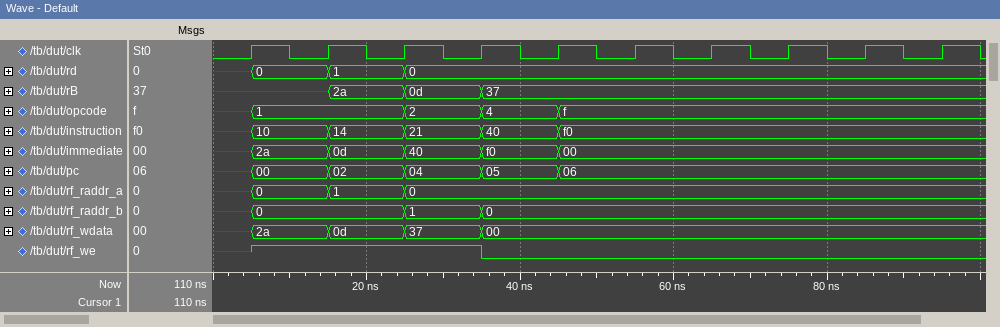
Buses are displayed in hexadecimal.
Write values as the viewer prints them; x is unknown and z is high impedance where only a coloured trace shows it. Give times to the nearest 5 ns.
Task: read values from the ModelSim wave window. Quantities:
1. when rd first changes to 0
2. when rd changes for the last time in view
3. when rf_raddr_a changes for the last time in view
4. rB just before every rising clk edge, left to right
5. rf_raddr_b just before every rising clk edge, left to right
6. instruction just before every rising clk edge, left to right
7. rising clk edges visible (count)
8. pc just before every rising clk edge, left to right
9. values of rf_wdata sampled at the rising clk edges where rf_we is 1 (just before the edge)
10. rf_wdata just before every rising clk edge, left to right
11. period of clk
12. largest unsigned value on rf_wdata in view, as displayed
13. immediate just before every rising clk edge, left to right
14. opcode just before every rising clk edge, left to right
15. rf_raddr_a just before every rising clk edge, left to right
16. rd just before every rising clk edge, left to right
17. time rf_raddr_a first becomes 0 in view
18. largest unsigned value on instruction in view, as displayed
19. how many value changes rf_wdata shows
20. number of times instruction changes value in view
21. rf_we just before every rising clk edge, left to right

5 ns
25 ns
25 ns
x, x, 2a, 0d, 37, 37, 37, 37, 37, 37
x, 0, 0, 1, 0, 0, 0, 0, 0, 0
x, 10, 14, 21, 40, f0, f0, f0, f0, f0
10
x, 00, 02, 04, 05, 06, 06, 06, 06, 06
2a, 0d, 37
x, 2a, 0d, 37, 00, 00, 00, 00, 00, 00
10 ns
37
x, 2a, 0d, 40, f0, 00, 00, 00, 00, 00
x, 1, 1, 2, 4, f, f, f, f, f
x, 0, 1, 0, 0, 0, 0, 0, 0, 0
x, 0, 1, 0, 0, 0, 0, 0, 0, 0
5 ns
f0
4
5
x 1 1 1 0 0 0 0 0 0
